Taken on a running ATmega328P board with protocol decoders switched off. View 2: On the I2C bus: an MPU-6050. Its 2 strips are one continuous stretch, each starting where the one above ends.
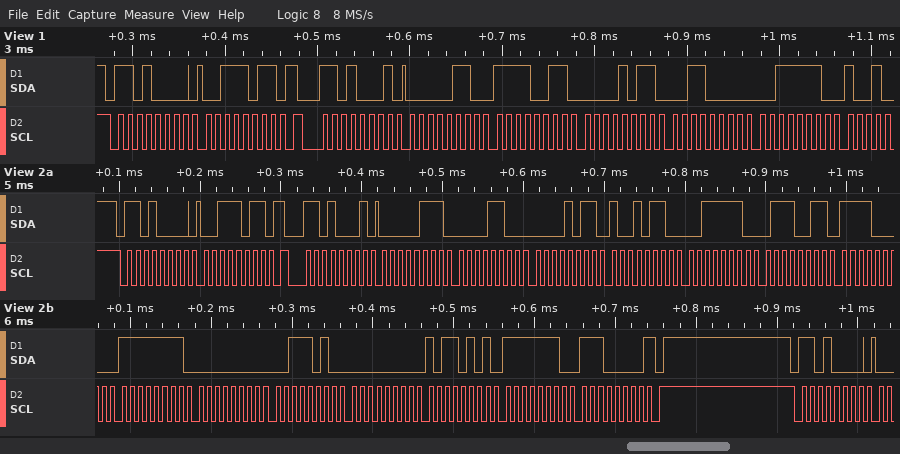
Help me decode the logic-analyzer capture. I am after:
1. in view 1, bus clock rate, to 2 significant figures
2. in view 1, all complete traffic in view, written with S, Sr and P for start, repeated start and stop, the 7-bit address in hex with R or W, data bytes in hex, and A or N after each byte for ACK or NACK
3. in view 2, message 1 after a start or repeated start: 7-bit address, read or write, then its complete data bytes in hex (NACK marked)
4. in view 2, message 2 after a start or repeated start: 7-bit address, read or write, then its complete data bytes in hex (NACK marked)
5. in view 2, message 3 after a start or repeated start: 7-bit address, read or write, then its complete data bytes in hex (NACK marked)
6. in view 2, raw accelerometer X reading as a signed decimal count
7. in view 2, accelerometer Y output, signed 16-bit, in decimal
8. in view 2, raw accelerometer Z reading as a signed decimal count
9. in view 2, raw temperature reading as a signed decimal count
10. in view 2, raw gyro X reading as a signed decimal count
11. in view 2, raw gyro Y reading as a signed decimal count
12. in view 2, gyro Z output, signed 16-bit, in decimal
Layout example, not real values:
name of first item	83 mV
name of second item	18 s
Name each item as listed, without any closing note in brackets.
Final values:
in view 1, bus clock rate, to 2 significant figures	100 kHz
in view 1, all complete traffic in view, written with S, Sr and P for start, repeated start and stop, the 7-bit address in hex with R or W, data bytes in hex, and A or N after each byte for ACK or NACK	S 68W A 3B A Sr 68R A 06 A F3 A 0B A 30 A 3E A
in view 2, message 1 after a start or repeated start: 7-bit address, read or write, then its complete data bytes in hex	0x68 write: 3B
in view 2, message 2 after a start or repeated start: 7-bit address, read or write, then its complete data bytes in hex	0x68 read: 07 0C 0B 96 3E 73 F0 FF 00 3A 00 B5 FE E0 NACK
in view 2, message 3 after a start or repeated start: 7-bit address, read or write, then its complete data bytes in hex	0x68 write
in view 2, raw accelerometer X reading as a signed decimal count	1804
in view 2, accelerometer Y output, signed 16-bit, in decimal	2966
in view 2, raw accelerometer Z reading as a signed decimal count	15987
in view 2, raw temperature reading as a signed decimal count	-3841
in view 2, raw gyro X reading as a signed decimal count	58
in view 2, raw gyro Y reading as a signed decimal count	181
in view 2, gyro Z output, signed 16-bit, in decimal	-288
